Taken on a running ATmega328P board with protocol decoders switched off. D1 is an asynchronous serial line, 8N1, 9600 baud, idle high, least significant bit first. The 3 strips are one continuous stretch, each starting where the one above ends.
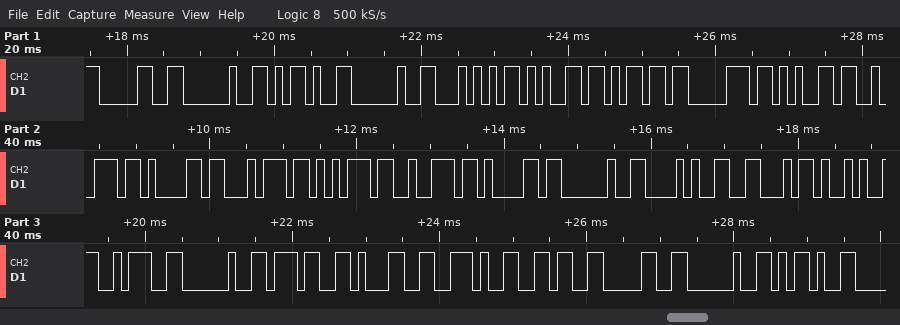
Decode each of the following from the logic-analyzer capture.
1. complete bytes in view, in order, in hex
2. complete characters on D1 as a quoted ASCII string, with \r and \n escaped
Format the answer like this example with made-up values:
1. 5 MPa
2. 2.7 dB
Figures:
1. 30 20 2D 20 54 65 6D 70 65 72 61 74 75 72 61 20 28 46 29 3A 20 37 31 2E 36 30 20 2D
2. "0 - Temperatura (F): 71.60 -"
